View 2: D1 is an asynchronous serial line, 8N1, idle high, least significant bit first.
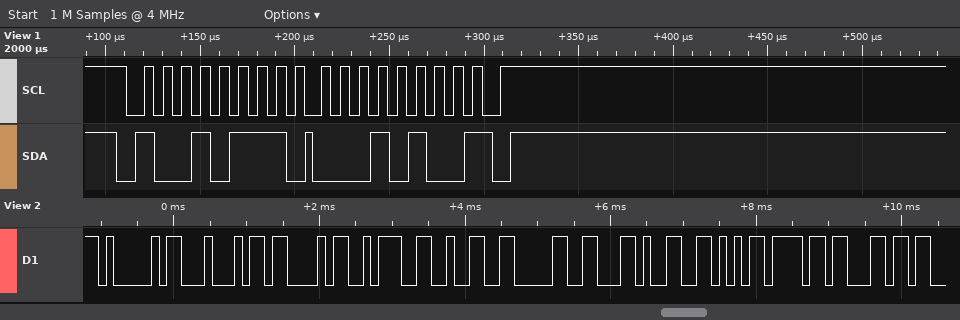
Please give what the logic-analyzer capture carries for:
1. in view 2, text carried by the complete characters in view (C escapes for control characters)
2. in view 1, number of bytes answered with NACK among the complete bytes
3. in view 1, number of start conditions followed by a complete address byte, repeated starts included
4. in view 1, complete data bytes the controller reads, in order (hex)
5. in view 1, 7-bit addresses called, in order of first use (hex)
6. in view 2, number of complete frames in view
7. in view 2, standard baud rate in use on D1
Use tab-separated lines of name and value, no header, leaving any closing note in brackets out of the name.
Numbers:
in view 2, text carried by the complete characters in view	"ADC:20,Vol"
in view 1, number of bytes answered with NACK among the complete bytes	1
in view 1, number of start conditions followed by a complete address byte, repeated starts included	1
in view 1, complete data bytes the controller reads, in order	14
in view 1, 7-bit addresses called, in order of first use	0x4B
in view 2, number of complete frames in view	10
in view 2, standard baud rate in use on D1	9600 baud
